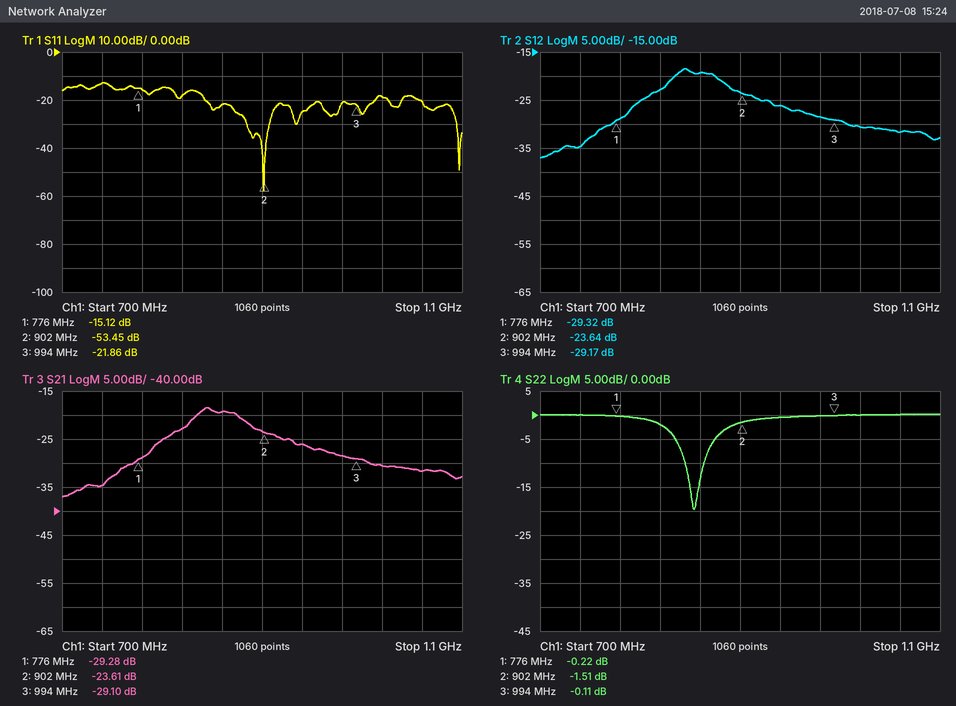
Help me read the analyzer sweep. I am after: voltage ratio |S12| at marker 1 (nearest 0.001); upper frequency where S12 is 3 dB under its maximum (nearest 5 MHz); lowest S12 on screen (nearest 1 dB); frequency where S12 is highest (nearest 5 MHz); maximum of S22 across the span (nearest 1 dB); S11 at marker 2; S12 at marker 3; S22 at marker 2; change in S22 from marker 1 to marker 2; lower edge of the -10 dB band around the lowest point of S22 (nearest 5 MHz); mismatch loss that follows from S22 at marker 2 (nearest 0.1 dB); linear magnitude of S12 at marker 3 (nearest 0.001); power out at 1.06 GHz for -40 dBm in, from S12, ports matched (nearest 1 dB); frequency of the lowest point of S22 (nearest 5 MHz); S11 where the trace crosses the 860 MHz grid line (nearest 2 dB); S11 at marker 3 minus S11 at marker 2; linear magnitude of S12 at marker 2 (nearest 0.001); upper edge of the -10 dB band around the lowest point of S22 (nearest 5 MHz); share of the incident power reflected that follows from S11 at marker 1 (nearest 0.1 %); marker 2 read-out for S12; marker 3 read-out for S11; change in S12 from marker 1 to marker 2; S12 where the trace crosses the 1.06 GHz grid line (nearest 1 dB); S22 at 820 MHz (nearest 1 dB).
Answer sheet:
0.034
885 MHz
-37 dB
845 MHz
0 dB
-53.45 dB
-29.17 dB
-1.51 dB
-1.29 dB
845 MHz
5.3 dB
0.035
-72 dBm
855 MHz
-22 dB
31.59 dB
0.066
865 MHz
3.1 %
-23.64 dB
-21.86 dB
5.68 dB
-32 dB
-2 dB
